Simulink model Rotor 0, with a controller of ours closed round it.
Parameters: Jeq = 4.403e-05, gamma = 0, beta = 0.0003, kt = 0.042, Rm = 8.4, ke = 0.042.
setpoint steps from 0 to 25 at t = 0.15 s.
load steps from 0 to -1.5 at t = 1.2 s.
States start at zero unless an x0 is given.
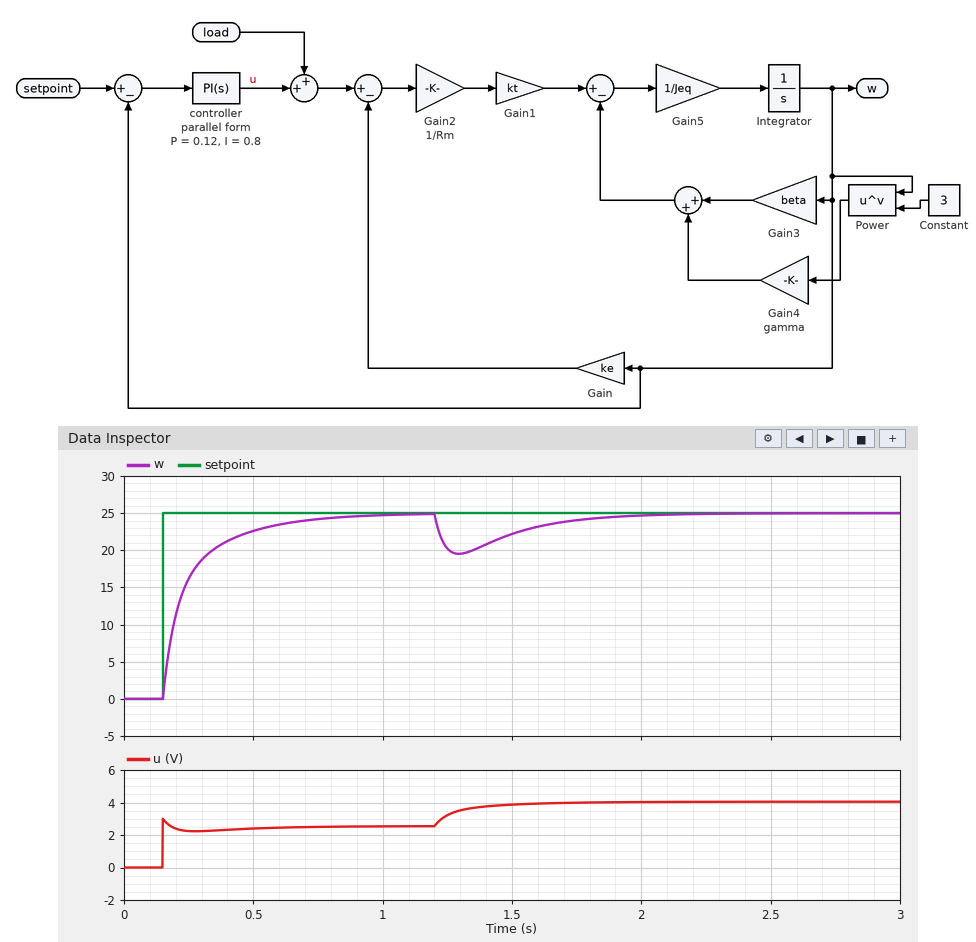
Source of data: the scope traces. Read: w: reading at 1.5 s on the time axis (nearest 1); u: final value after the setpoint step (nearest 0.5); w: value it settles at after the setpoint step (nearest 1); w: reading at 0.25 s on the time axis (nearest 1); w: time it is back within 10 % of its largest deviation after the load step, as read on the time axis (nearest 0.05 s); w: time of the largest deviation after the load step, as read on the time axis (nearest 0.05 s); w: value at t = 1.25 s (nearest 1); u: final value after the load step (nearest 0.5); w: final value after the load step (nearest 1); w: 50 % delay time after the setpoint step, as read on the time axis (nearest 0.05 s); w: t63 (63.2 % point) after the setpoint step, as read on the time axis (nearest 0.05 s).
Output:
22
2.5
25
16
1.90 s
1.30 s
20
4.0
25
0.20 s
0.25 s
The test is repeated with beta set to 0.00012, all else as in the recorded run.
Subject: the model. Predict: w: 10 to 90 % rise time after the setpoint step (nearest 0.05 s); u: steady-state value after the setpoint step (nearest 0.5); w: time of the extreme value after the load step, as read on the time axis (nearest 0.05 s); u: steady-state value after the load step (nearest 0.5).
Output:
0.20 s
1.5
1.30 s
3.0
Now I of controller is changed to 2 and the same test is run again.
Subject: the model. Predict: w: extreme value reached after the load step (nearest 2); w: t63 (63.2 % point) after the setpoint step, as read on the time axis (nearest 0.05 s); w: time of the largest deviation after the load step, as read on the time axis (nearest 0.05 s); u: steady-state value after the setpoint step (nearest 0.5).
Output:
20
0.20 s
1.25 s
2.5
